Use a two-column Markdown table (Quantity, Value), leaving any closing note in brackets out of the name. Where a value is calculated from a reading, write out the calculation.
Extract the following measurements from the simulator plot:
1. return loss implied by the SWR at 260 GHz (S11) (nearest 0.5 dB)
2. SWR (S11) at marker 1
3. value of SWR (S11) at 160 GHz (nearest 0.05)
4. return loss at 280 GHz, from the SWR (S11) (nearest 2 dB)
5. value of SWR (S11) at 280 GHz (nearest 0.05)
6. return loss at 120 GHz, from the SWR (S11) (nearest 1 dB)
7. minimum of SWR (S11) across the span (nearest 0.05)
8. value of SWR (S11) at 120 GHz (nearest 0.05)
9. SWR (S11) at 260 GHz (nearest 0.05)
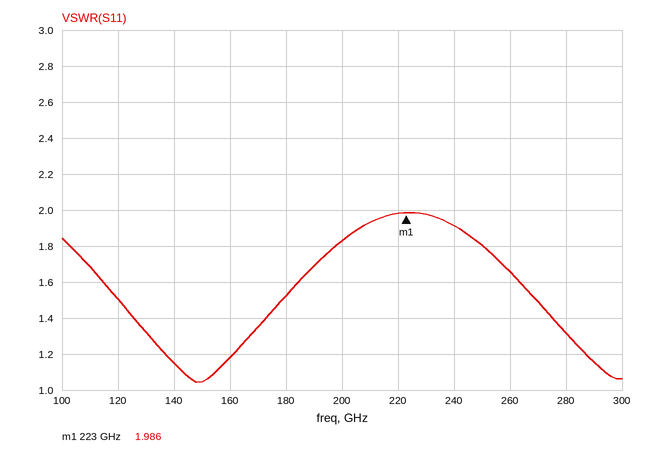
| Quantity | Value |
|---|---|
| return loss implied by the SWR at 260 GHz (S11) | −20 log10((1.65 − 1)/(1.65 + 1)) ≈ 12.2 dB, so 12.0 dB to the nearest 0.5 dB |
| SWR (S11) at marker 1 | 1.986 |
| value of SWR (S11) at 160 GHz | 1.20 |
| return loss at 280 GHz, from the SWR (S11) | −20 log10((1.3 − 1)/(1.3 + 1)) ≈ 18 dB |
| value of SWR (S11) at 280 GHz | 1.30 |
| return loss at 120 GHz, from the SWR (S11) | −20 log10((1.5 − 1)/(1.5 + 1)) ≈ 14 dB |
| minimum of SWR (S11) across the span | 1.05 |
| value of SWR (S11) at 120 GHz | 1.50 |
| SWR (S11) at 260 GHz | 1.65 |
